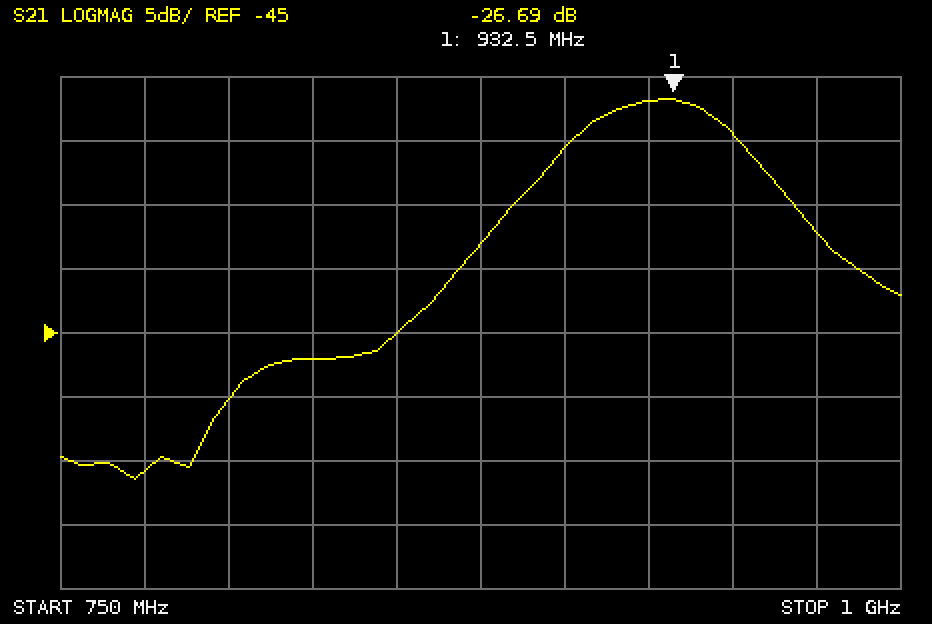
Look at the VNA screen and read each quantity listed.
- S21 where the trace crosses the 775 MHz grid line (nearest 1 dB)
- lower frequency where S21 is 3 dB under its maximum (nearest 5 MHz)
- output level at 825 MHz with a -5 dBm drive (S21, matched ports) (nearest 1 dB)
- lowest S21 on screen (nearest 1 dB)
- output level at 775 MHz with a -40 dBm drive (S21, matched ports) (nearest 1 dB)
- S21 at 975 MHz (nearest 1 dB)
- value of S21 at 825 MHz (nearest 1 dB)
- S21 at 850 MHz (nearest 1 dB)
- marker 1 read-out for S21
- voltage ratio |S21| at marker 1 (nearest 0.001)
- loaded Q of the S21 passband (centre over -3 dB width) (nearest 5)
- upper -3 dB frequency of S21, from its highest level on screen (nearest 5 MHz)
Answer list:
-56 dB
905 MHz
-52 dBm
-56 dB
-96 dBm
-37 dB
-47 dB
-45 dB
-26.69 dB
0.046
20
950 MHz
